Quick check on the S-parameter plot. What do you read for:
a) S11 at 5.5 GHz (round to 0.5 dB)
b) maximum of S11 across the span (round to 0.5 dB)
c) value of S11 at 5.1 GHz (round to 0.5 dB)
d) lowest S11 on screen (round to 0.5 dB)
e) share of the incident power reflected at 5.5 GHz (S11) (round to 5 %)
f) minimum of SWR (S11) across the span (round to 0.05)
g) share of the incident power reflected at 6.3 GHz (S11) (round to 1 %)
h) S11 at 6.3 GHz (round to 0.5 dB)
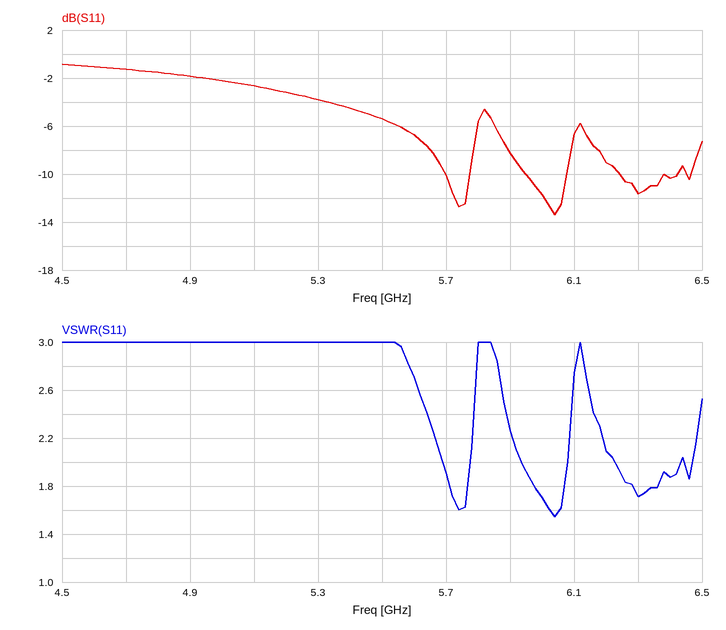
-5.5 dB
-1.0 dB
-2.5 dB
-13.5 dB
30 %
1.55
7 %
-11.5 dB
